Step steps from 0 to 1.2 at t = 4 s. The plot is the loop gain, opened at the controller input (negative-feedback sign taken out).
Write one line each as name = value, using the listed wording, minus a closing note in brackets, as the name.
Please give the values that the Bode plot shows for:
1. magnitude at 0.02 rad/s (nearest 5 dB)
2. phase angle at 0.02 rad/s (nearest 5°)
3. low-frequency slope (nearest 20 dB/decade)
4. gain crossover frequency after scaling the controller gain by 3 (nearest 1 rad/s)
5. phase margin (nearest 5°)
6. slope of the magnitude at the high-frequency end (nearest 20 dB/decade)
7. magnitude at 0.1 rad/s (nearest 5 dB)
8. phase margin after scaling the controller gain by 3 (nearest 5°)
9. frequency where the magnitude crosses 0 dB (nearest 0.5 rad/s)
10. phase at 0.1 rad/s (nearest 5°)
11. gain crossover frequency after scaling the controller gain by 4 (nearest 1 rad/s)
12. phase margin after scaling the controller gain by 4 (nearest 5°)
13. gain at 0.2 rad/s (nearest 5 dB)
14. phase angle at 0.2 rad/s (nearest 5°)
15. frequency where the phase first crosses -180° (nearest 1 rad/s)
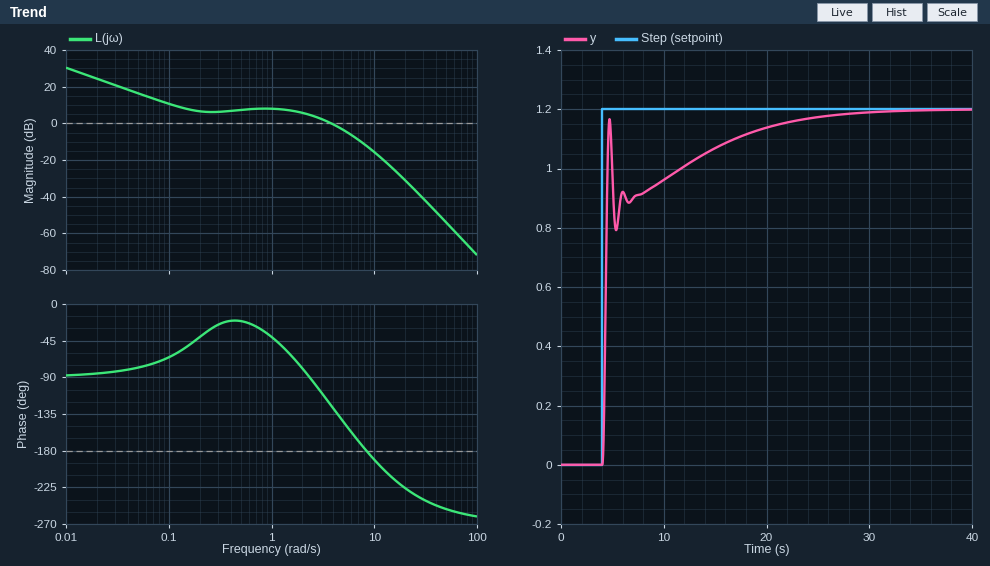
magnitude at 0.02 rad/s = 25 dB
phase angle at 0.02 rad/s = -85°
low-frequency slope = -20 dB/decade
gain crossover frequency after scaling the controller gain by 3 = 7 rad/s
phase margin = 55°
slope of the magnitude at the high-frequency end = -60 dB/decade
magnitude at 0.1 rad/s = 10 dB
phase margin after scaling the controller gain by 3 = 10°
frequency where the magnitude crosses 0 dB = 4.0 rad/s
phase at 0.1 rad/s = -65°
gain crossover frequency after scaling the controller gain by 4 = 8 rad/s
phase margin after scaling the controller gain by 4 = 0°
gain at 0.2 rad/s = 5 dB
phase angle at 0.2 rad/s = -40°
frequency where the phase first crosses -180° = 8 rad/s
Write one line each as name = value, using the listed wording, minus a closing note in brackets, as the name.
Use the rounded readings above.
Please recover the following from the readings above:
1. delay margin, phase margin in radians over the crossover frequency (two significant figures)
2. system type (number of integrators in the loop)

delay margin, phase margin in radians over the crossover frequency = 0.24 s
system type = 1
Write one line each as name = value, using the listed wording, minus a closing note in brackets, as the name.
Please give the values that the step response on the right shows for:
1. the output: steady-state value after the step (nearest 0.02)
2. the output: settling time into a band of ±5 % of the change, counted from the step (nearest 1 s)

the output: steady-state value after the step = 1.20
the output: settling time into a band of ±5 % of the change, counted from the step = 16 s
